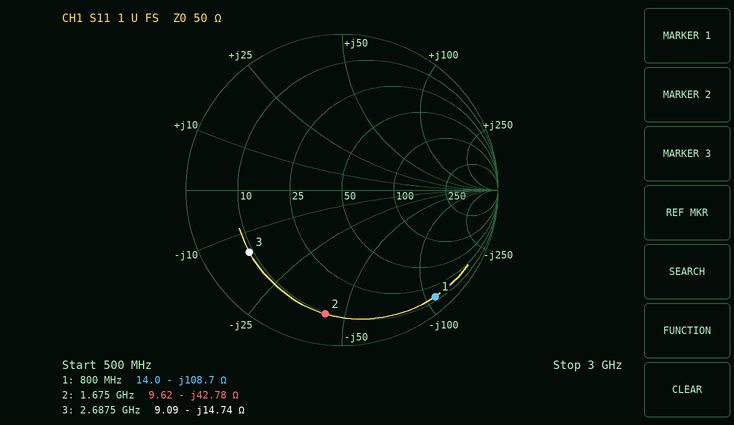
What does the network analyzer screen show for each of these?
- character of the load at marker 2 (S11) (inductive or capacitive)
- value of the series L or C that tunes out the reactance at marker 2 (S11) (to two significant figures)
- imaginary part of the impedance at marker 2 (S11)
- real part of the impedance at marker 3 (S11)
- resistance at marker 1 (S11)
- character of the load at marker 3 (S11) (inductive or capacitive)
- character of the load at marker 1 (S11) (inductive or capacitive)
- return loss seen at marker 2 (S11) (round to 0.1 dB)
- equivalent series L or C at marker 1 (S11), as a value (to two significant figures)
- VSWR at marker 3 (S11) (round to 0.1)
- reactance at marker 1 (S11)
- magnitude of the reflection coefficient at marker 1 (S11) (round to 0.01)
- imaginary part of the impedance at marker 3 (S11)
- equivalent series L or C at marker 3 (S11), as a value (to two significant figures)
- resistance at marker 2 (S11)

capacitive
4.1 nH
-42.78 Ω
9.09 Ω
14.0 Ω
capacitive
capacitive
1.9 dB
1.8 pF
6.0
-108.7 Ω
0.91
-14.74 Ω
4.0 pF
9.62 Ω
